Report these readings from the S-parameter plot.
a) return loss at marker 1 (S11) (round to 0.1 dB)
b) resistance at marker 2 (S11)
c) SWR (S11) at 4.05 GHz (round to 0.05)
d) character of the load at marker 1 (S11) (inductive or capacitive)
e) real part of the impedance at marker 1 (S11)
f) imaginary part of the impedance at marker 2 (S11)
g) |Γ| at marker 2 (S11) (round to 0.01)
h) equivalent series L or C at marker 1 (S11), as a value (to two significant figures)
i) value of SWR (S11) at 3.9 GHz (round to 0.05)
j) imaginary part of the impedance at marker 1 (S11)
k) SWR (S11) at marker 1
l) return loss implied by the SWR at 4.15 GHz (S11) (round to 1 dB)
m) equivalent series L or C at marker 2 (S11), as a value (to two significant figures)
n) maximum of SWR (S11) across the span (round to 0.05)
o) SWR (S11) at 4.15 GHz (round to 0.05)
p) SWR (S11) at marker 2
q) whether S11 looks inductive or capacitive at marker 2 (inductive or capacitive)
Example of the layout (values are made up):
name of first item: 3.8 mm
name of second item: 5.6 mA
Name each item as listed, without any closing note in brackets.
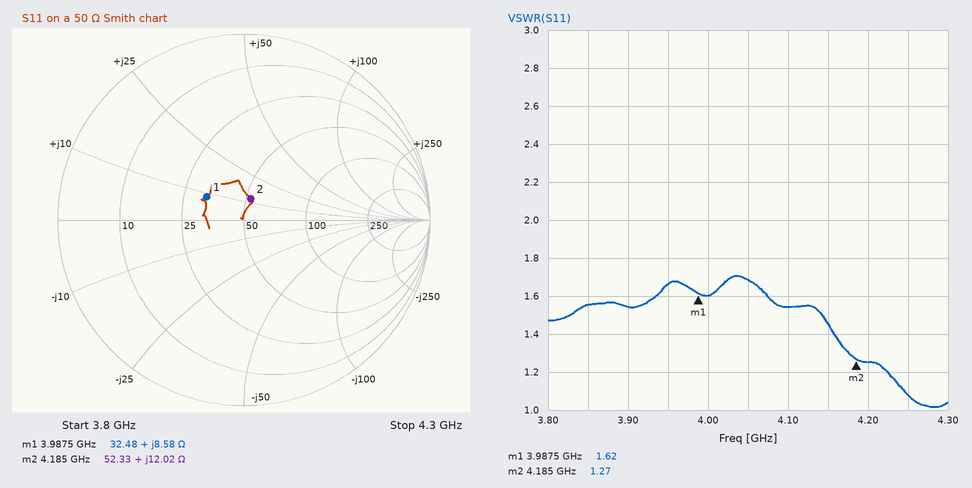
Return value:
return loss at marker 1 (S11): 12.6 dB
resistance at marker 2: 52.33 Ω
SWR (S11) at 4.05 GHz: 1.70
character of the load at marker 1 (S11): inductive
real part of the impedance at marker 1: 32.48 Ω
imaginary part of the impedance at marker 2: +12.02 Ω
|Γ| at marker 2 (S11): 0.12
equivalent series L or C at marker 1 (S11), as a value: 340 pH
value of SWR (S11) at 3.9 GHz: 1.55
imaginary part of the impedance at marker 1: +8.58 Ω
SWR (S11) at marker 1: 1.62
return loss implied by the SWR at 4.15 GHz (S11): 15 dB
equivalent series L or C at marker 2 (S11), as a value: 460 pH
maximum of SWR (S11) across the span: 1.70
SWR (S11) at 4.15 GHz: 1.45
SWR (S11) at marker 2: 1.27
whether S11 looks inductive or capacitive at marker 2: inductive
